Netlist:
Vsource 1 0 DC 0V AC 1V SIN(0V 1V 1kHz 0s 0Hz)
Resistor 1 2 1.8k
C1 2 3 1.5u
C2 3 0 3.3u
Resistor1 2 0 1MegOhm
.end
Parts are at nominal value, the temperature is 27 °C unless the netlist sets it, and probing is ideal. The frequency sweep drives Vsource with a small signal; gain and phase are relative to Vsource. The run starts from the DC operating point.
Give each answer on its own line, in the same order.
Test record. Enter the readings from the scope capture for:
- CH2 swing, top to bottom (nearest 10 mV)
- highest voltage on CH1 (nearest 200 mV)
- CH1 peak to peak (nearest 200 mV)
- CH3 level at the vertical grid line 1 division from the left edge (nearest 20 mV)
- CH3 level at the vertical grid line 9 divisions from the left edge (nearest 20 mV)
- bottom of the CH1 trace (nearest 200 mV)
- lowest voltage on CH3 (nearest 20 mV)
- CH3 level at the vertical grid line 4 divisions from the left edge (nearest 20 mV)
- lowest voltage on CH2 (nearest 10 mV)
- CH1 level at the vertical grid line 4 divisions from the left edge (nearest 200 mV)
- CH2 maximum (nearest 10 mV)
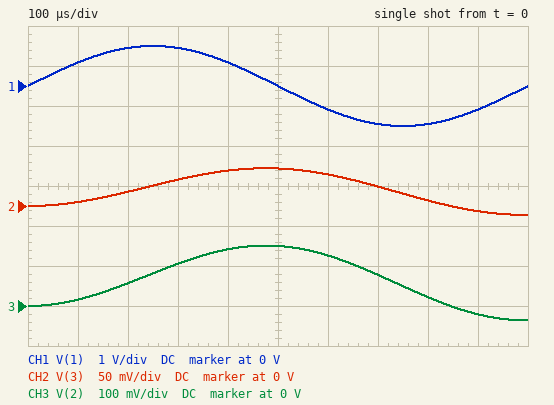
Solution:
60 mV
1.0 V
2.0 V
20 mV
-20 mV
-1.0 V
-40 mV
140 mV
-10 mV
600 mV
50 mV
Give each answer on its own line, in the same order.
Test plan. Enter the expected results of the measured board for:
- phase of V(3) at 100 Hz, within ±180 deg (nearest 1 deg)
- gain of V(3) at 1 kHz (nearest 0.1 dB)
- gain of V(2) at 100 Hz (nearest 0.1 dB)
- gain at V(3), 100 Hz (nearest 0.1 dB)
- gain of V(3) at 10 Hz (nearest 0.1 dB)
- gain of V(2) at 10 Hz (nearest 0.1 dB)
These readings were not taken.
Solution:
-49 deg
-31.5 dB
-3.7 dB
-13.8 dB
-10.2 dB
-0.1 dB
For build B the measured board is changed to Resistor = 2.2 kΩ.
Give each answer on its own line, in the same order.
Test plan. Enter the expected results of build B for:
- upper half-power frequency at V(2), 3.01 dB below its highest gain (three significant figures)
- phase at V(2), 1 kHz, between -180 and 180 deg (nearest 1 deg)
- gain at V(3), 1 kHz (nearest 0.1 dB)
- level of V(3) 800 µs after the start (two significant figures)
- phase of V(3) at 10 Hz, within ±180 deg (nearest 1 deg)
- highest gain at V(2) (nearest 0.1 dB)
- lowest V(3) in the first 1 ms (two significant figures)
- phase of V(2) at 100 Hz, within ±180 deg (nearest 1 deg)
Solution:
70.3 Hz
-86 deg
-33.2 dB
7.1 mV
-8 deg
0 dB
-7.8 mV
-55 deg
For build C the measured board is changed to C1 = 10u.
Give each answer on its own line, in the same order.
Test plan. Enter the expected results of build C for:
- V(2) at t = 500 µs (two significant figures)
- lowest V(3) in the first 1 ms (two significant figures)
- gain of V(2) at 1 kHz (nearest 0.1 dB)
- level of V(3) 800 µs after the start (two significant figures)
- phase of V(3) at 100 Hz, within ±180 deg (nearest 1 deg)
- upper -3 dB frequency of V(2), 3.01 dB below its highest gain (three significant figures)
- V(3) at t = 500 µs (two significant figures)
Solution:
67 mV
-5.4 mV
-29.0 dB
13 mV
-70 deg
35.7 Hz
51 mV
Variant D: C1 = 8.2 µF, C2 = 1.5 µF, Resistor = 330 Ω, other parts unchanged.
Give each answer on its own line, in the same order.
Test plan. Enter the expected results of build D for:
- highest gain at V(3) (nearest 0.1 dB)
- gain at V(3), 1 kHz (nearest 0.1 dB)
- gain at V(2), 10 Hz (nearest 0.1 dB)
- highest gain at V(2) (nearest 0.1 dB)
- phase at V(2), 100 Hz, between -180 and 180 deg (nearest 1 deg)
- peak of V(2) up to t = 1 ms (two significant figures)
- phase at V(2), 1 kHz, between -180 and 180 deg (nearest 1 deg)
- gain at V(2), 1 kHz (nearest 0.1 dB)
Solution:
-1.5 dB
-10.4 dB
0 dB
0 dB
-15 deg
470 mV
-69 deg
-9.0 dB
